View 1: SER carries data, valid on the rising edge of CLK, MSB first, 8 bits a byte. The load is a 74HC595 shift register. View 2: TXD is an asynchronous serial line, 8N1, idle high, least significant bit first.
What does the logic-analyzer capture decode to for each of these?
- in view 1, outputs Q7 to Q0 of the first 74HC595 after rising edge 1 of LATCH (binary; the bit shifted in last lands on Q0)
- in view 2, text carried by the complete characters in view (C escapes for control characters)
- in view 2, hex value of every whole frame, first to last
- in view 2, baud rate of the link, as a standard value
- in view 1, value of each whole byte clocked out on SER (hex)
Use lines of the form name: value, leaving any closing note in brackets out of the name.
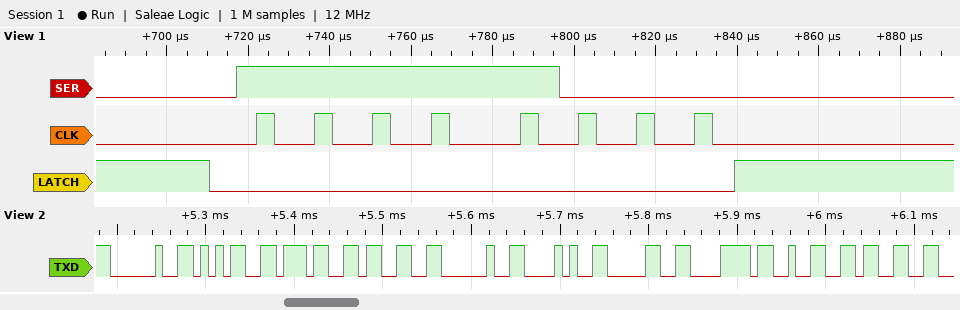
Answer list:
in view 1, outputs Q7 to Q0 of the first 74HC595 after rising edge 1 of LATCH: 11111000
in view 2, text carried by the complete characters in view: " 573 (0x23"
in view 2, hex value of every whole frame, first to last: 0x20 0x35 0x37 0x33 0x20 0x28 0x30 0x78 0x32 0x33
in view 2, baud rate of the link, as a standard value: 115200 baud
in view 1, value of each whole byte clocked out on SER: F8
